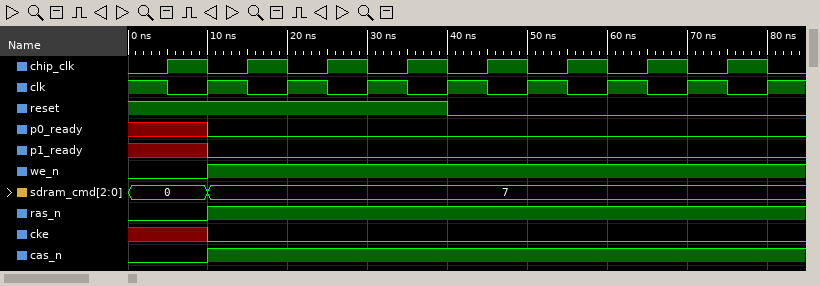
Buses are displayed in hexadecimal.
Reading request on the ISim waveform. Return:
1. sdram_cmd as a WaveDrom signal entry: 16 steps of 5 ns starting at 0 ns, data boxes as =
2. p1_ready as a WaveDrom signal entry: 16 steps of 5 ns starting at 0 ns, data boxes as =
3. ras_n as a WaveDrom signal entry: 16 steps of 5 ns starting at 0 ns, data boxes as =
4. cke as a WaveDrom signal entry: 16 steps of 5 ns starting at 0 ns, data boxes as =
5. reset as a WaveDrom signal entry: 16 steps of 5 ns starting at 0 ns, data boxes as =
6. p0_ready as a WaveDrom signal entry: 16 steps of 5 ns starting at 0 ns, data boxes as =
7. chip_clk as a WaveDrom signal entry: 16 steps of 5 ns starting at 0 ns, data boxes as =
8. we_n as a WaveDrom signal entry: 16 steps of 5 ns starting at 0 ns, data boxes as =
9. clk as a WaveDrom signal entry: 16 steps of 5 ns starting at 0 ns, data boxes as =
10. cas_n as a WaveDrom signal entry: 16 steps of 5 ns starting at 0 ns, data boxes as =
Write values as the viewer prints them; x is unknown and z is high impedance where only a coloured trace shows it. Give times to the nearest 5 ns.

{name: 'sdram_cmd', wave: '=.=.............', data: '0 7'}
{name: 'p1_ready', wave: 'x.0.............'}
{name: 'ras_n', wave: '0.1.............'}
{name: 'cke', wave: 'x.0.............'}
{name: 'reset', wave: '1.......0.......'}
{name: 'p0_ready', wave: 'x.0.............'}
{name: 'chip_clk', wave: '0101010101010101'}
{name: 'we_n', wave: '0.1.............'}
{name: 'clk', wave: '1010101010101010'}
{name: 'cas_n', wave: '0.1.............'}
